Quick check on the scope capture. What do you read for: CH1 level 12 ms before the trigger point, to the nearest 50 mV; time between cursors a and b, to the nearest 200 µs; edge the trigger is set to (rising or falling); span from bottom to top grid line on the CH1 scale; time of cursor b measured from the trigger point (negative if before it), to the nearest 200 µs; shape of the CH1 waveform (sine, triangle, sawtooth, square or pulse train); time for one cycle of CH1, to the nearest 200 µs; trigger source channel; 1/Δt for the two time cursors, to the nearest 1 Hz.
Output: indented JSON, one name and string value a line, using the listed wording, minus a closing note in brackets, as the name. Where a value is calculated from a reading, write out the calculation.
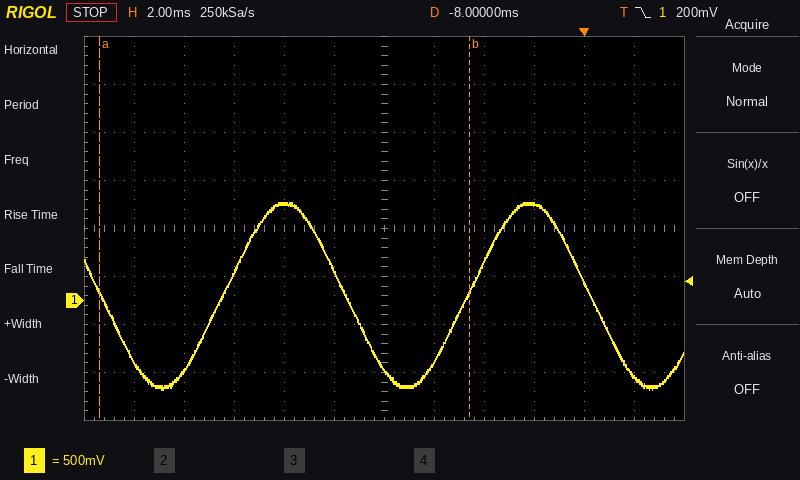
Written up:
{
  "CH1 level 12 ms before the trigger point, to the nearest 50 mV": "1.00 V",
  "time between cursors a and b, to the nearest 200 µs": "14.8 ms",
  "edge the trigger is set to": "falling",
  "span from bottom to top grid line on the CH1 scale": "4 V",
  "time of cursor b measured from the trigger point (negative if before it), to the nearest 200 µs": "-4.6 ms",
  "shape of the CH1 waveform": "sine",
  "time for one cycle of CH1, to the nearest 200 µs": "9.8 ms",
  "trigger source channel": "CH1",
  "1/Δt for the two time cursors, to the nearest 1 Hz": "1 / 14.8 ms ≈ 68 Hz"
}
